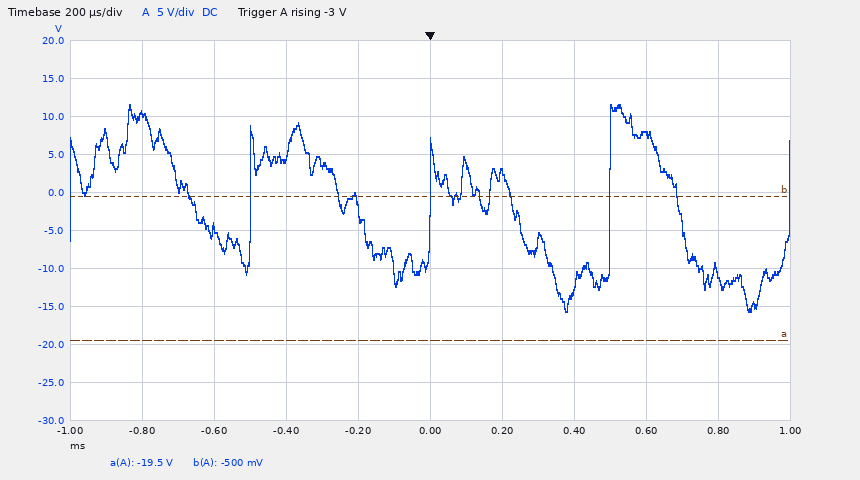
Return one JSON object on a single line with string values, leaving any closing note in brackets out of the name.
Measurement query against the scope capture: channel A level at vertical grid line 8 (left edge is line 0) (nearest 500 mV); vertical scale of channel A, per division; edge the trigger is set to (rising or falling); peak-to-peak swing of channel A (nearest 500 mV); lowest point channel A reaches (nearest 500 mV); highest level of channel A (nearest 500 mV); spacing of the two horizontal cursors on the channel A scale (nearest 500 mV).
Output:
{"channel A level at vertical grid line 8 (left edge is line 0)": "7.5 V", "vertical scale of channel A, per division": "5 V", "edge the trigger is set to": "rising", "peak-to-peak swing of channel A": "27.0 V", "lowest point channel A reaches": "-15.5 V", "highest level of channel A": "11.5 V", "spacing of the two horizontal cursors on the channel A scale": "19.0 V"}
